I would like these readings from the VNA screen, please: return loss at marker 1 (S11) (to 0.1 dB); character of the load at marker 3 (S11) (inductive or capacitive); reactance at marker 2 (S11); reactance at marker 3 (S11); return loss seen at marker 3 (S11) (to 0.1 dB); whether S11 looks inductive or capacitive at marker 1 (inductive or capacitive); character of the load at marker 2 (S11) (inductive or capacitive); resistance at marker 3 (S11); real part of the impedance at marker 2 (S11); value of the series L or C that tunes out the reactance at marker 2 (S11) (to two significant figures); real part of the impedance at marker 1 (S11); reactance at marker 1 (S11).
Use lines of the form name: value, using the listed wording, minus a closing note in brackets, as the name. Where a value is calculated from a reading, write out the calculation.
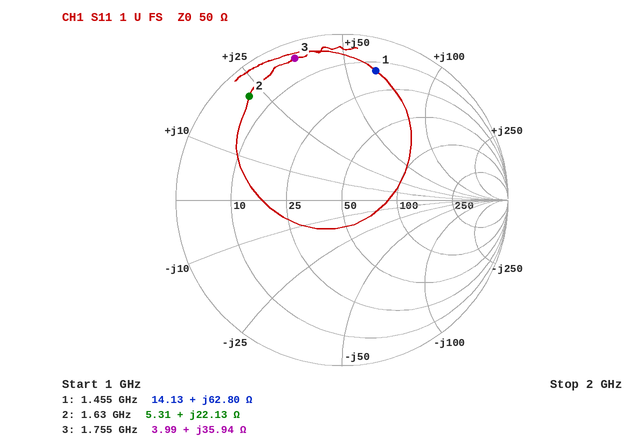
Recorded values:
return loss at marker 1 (S11): 1.9 dB
character of the load at marker 3 (S11): inductive
reactance at marker 2: +22.13 Ω
reactance at marker 3: +35.94 Ω
return loss seen at marker 3 (S11): 0.9 dB
whether S11 looks inductive or capacitive at marker 1: inductive
character of the load at marker 2 (S11): inductive
resistance at marker 3: 3.99 Ω
real part of the impedance at marker 2: 5.31 Ω
value of the series L or C that tunes out the reactance at marker 2 (S11): C = 1/(2π × 1.63 GHz × 22.13 Ω) ≈ 4.4 pF
real part of the impedance at marker 1: 14.13 Ω
reactance at marker 1: +62.80 Ω
